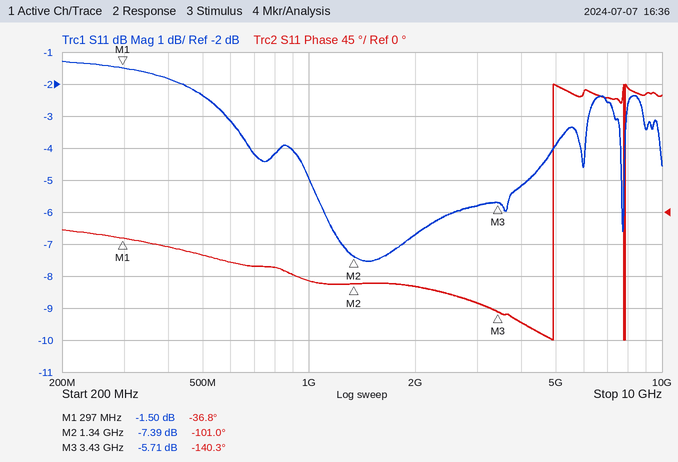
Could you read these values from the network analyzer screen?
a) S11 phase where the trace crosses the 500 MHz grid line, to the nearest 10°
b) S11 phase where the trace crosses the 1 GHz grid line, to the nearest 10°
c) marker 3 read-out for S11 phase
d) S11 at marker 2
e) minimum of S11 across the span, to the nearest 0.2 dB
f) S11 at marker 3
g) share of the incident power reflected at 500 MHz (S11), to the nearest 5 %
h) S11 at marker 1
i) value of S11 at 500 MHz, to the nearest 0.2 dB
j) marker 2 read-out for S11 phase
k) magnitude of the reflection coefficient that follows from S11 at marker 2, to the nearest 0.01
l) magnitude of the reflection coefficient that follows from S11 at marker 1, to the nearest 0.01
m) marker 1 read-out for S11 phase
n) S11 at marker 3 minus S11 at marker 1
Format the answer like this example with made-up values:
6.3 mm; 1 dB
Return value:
-60°; -100°; -140.3°; -7.39 dB; -7.6 dB; -5.71 dB; 60 %; -1.50 dB; -2.4 dB; -101.0°; 0.43; 0.84; -36.8°; -4.21 dB
